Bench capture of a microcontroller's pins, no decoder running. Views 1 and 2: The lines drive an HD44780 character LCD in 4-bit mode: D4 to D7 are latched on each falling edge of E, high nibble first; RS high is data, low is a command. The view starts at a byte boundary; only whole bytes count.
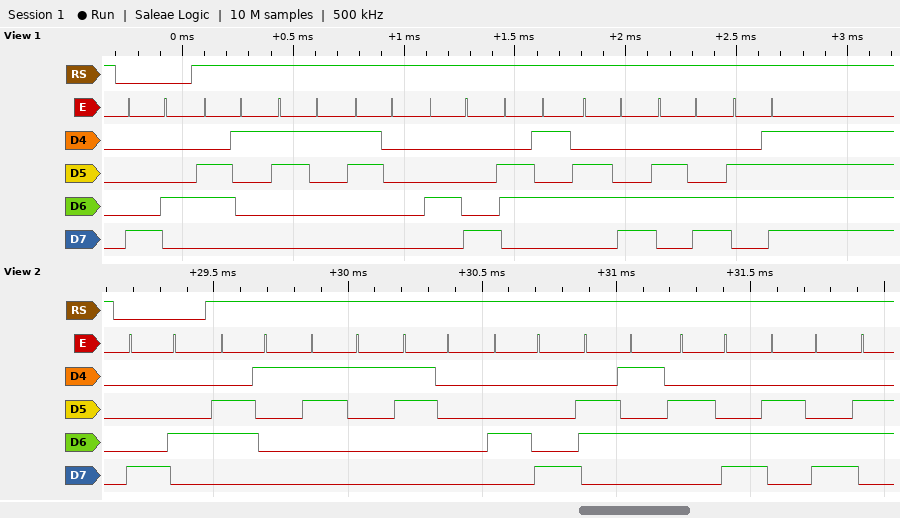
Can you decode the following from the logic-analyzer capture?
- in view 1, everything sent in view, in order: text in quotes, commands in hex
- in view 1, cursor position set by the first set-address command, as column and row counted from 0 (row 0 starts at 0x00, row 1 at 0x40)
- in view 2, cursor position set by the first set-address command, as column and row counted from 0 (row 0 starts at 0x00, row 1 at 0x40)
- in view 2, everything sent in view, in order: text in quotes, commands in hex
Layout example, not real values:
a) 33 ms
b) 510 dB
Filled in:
a) 0x84 "a10Hello"
b) column 4, row 0
c) column 4, row 0
d) 0x84 "a10Hell"
